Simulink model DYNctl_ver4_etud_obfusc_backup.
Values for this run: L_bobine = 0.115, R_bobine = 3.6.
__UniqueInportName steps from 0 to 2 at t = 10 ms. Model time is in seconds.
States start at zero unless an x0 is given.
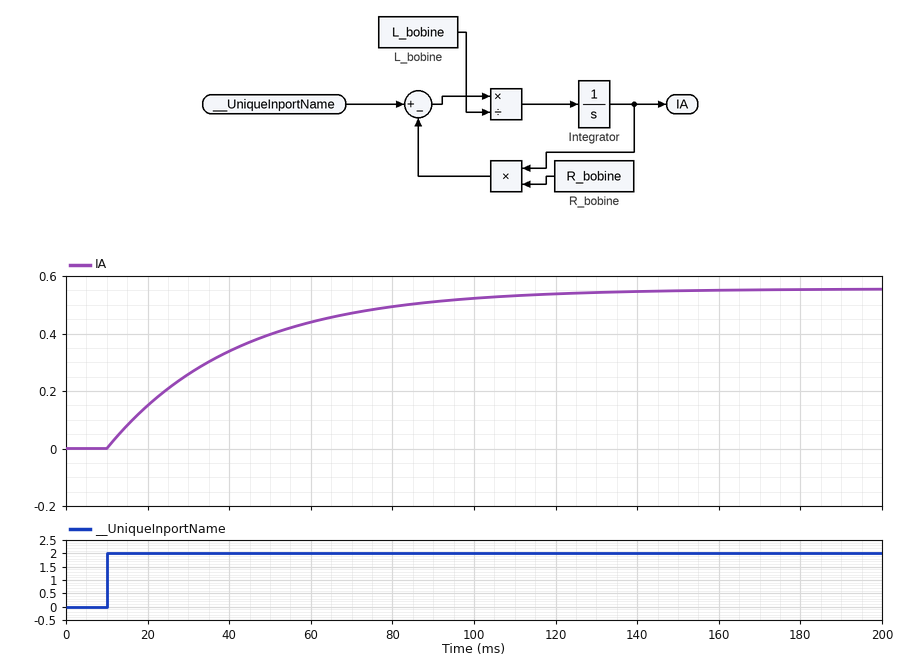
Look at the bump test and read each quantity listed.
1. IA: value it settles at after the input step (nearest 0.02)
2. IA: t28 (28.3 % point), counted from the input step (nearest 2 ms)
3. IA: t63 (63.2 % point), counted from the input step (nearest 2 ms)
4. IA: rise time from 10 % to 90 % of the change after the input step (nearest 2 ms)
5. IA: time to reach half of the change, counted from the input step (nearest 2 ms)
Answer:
0.56
10 ms
32 ms
70 ms
22 ms
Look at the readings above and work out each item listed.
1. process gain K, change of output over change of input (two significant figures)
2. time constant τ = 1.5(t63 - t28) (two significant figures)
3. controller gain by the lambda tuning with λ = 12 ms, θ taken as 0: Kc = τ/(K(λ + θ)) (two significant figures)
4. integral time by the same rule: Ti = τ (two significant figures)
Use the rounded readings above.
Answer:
0.28
33 ms
9.8
33 ms
